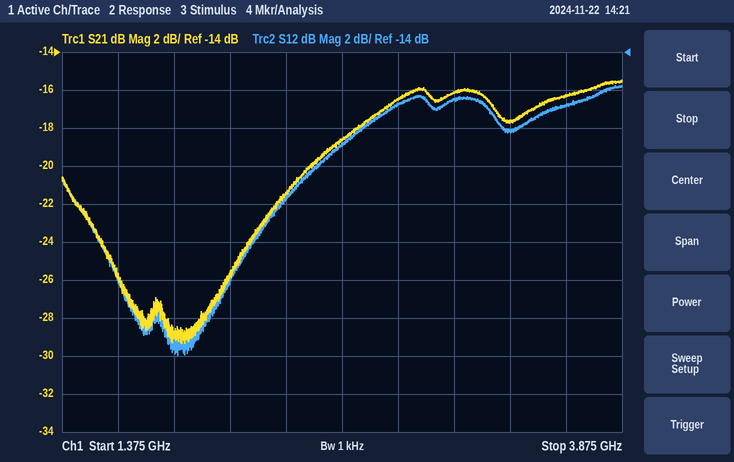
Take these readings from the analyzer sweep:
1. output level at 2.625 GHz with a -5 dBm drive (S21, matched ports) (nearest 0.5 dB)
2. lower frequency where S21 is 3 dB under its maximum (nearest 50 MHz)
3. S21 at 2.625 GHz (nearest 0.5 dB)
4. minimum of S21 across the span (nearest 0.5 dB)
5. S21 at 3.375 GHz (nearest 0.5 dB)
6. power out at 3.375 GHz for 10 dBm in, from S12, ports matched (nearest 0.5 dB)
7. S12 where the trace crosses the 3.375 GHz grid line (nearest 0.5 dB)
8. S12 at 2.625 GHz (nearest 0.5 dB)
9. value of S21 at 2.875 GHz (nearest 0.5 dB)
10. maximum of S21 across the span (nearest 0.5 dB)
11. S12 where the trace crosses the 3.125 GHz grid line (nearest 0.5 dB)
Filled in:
-23.5 dBm
2.65 GHz
-18.5 dB
-29.5 dB
-17.5 dB
-8.0 dBm
-18.0 dB
-19.0 dB
-16.5 dB
-15.5 dB
-16.5 dB
